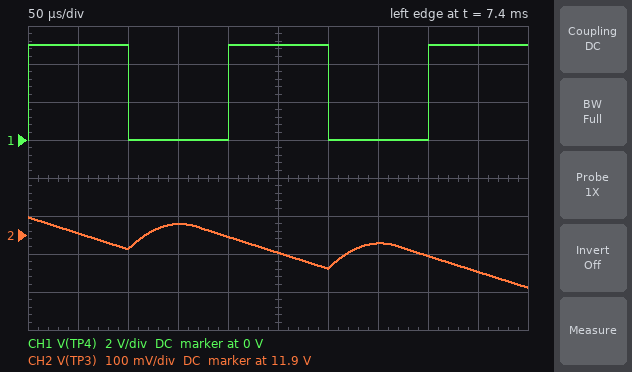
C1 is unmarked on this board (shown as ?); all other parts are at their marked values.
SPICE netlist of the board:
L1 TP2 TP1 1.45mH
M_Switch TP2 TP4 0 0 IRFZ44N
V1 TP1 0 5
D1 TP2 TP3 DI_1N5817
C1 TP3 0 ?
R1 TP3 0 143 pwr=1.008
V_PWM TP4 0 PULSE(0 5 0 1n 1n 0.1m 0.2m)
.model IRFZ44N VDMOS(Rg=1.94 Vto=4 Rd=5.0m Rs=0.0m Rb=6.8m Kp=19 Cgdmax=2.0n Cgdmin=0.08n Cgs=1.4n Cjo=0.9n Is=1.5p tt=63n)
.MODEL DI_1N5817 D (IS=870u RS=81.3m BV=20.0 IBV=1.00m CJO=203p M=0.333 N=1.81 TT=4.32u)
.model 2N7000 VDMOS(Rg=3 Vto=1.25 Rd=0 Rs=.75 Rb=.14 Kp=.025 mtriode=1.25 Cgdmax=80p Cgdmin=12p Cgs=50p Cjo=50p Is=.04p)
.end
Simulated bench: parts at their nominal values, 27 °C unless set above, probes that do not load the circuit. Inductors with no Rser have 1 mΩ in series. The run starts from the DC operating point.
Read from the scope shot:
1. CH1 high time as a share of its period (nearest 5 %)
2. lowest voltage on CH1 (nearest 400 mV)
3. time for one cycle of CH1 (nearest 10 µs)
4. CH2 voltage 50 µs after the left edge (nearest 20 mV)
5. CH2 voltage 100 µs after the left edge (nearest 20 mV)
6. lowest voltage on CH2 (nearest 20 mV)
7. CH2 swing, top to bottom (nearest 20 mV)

50 %
0 V
200 µs
11.90 V
11.86 V
11.76 V
180 mV
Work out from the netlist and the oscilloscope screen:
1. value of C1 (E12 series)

100 µF
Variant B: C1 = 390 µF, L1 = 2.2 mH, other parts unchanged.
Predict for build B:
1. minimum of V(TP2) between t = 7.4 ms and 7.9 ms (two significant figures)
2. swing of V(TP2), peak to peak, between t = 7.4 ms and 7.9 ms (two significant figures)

-620 mV
14 V
